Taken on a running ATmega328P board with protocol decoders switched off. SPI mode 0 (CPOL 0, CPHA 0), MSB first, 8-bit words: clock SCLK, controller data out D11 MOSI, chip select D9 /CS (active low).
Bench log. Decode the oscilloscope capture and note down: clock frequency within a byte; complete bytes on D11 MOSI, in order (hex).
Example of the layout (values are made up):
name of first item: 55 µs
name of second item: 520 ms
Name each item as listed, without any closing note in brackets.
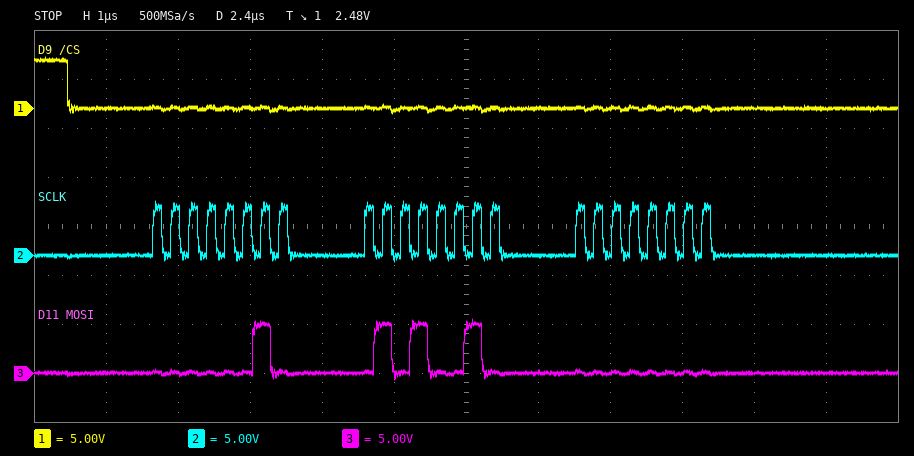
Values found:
clock frequency within a byte: 4 MHz
complete bytes on D11 MOSI, in order: 02 52 00
